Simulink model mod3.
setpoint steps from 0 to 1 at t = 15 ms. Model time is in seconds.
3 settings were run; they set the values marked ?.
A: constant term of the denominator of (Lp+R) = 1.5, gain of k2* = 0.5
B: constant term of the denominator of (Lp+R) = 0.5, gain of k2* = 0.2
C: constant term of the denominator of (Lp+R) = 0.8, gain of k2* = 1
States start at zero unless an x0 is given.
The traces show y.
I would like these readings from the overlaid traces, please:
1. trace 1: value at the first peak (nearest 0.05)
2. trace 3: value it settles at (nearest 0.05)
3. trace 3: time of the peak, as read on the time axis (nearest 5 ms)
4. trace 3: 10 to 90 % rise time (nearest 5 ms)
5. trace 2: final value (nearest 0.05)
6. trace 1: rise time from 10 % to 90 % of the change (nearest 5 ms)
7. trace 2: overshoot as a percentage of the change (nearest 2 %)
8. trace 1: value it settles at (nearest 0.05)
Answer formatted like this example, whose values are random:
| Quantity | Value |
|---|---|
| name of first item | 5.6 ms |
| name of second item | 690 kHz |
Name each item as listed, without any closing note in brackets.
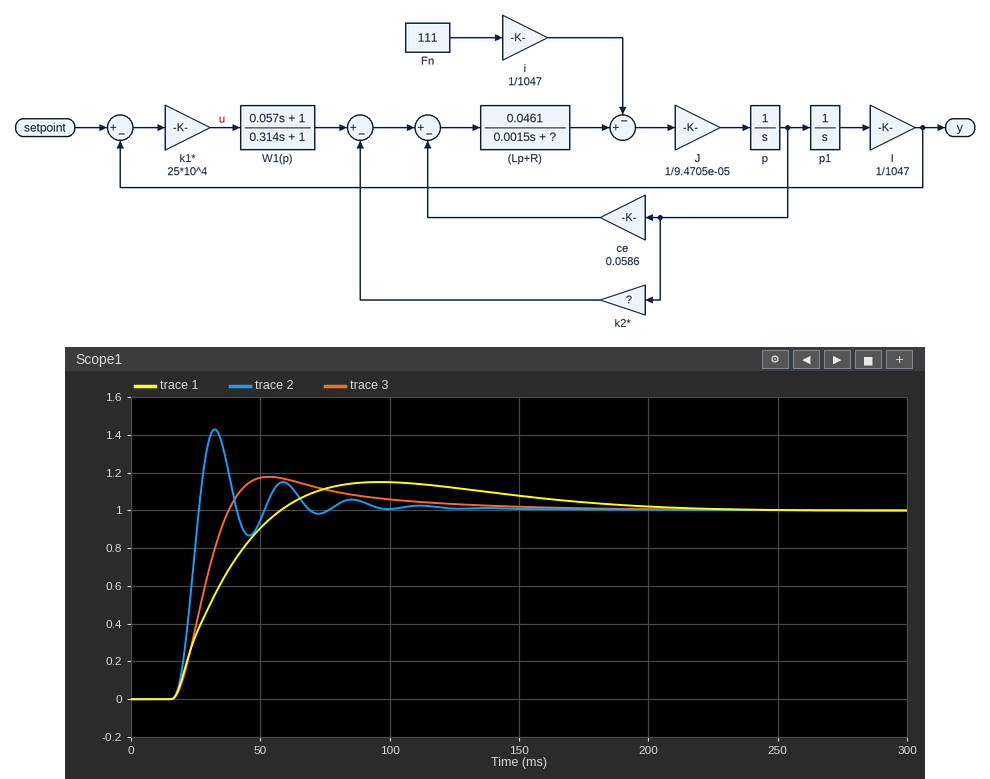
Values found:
| Quantity | Value |
|---|---|
| trace 1: value at the first peak | 1.15 |
| trace 3: value it settles at | 1.00 |
| trace 3: time of the peak, as read on the time axis | 55 ms |
| trace 3: 10 to 90 % rise time | 15 ms |
| trace 2: final value | 1.00 |
| trace 1: rise time from 10 % to 90 % of the change | 30 ms |
| trace 2: overshoot as a percentage of the change | 42 % |
| trace 1: value it settles at | 1.00 |
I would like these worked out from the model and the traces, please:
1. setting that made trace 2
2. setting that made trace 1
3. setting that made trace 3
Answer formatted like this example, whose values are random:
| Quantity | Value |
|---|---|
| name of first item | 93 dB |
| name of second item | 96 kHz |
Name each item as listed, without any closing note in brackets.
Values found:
| Quantity | Value |
|---|---|
| setting that made trace 2 | B |
| setting that made trace 1 | C |
| setting that made trace 3 | A |
